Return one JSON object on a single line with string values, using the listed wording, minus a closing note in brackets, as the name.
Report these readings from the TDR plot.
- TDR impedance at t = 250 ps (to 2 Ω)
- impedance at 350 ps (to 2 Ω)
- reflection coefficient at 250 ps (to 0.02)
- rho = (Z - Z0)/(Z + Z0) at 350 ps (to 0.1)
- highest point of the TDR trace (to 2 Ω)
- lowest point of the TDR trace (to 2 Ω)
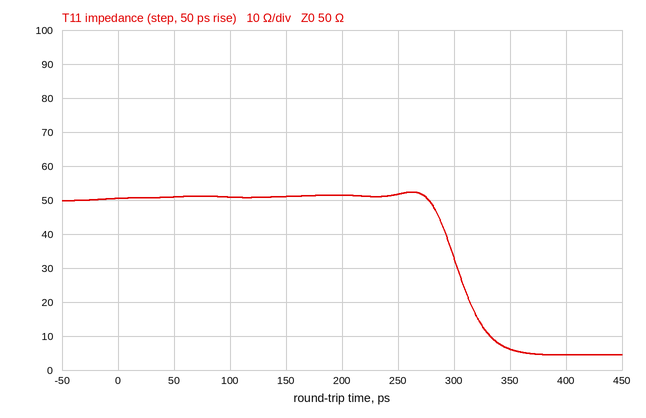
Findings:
{"TDR impedance at t = 250 ps": "52 Ω", "impedance at 350 ps": "6 Ω", "reflection coefficient at 250 ps": "+0.02", "rho = (Z - Z0)/(Z + Z0) at 350 ps": "-0.8", "highest point of the TDR trace": "52 Ω", "lowest point of the TDR trace": "4 Ω"}
